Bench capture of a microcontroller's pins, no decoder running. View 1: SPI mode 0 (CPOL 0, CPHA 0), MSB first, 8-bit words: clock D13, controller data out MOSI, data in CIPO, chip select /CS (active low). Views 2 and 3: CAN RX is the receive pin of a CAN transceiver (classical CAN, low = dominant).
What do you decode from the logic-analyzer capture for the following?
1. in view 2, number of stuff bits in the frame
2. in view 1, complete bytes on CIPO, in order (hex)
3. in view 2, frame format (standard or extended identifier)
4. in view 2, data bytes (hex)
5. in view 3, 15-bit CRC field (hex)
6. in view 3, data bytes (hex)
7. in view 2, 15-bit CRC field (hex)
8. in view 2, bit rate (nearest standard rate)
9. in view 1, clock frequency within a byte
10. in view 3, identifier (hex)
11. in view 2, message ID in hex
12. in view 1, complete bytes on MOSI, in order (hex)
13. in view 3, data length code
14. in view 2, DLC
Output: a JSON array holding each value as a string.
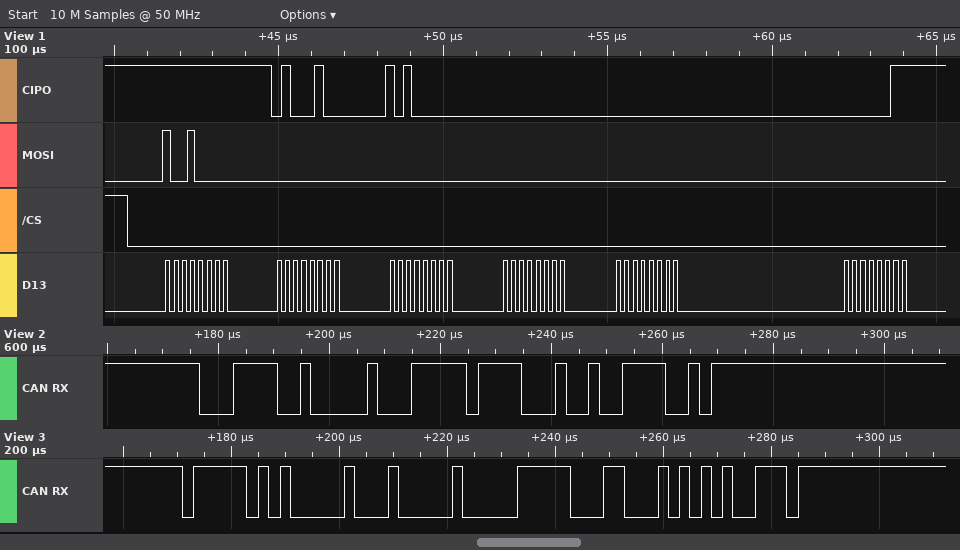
["2", "0xFF 0x44 0xA0 0x00 0x00 0x03", "standard", "FF", "0x4553", "00 79", "0x093C", "500 kbit/s", "4 MHz", "0x7E8", "0x1E4", "0x90 0x00 0x00 0x00 0x00 0x00", "2", "1"]
